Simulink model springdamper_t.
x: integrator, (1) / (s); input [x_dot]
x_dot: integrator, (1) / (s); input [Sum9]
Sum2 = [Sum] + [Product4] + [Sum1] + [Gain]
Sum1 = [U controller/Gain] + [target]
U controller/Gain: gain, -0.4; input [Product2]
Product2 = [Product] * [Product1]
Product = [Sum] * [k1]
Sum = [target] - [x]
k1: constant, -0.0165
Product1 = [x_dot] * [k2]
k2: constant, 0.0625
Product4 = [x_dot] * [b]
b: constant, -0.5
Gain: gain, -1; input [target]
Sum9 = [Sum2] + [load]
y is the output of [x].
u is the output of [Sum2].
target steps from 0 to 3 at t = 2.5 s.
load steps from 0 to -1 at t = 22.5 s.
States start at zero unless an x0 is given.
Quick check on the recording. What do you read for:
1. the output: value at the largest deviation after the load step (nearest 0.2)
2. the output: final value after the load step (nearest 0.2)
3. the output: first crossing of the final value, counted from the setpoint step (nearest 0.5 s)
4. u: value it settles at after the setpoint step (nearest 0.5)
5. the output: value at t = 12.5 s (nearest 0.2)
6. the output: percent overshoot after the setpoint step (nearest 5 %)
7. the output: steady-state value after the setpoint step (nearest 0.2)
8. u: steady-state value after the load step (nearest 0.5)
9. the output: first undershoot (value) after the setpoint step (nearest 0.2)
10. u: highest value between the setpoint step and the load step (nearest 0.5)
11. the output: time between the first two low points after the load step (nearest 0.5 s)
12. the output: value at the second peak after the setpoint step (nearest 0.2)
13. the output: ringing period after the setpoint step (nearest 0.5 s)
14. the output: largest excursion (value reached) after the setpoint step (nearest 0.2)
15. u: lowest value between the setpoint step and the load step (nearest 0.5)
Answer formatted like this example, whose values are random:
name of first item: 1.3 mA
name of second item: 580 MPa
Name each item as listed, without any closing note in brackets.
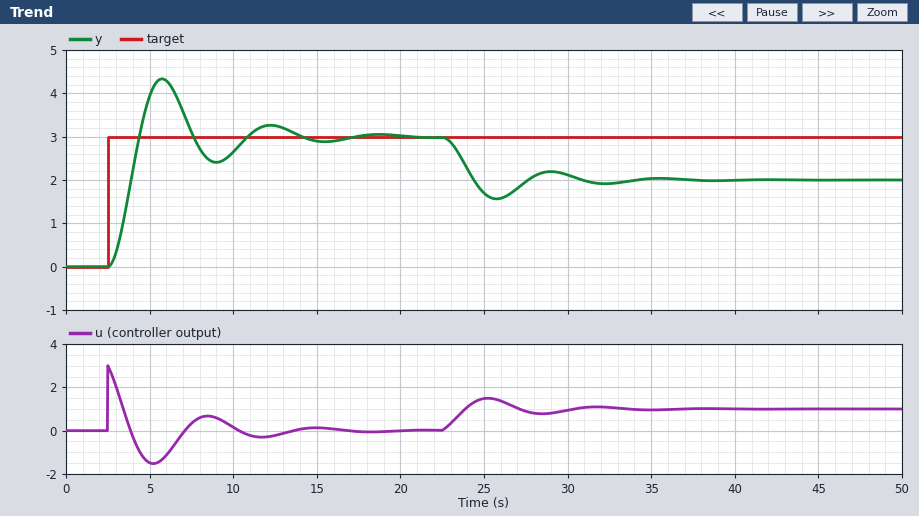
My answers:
the output: value at the largest deviation after the load step: 1.6
the output: final value after the load step: 2.0
the output: first crossing of the final value, counted from the setpoint step: 2.0 s
u: value it settles at after the setpoint step: 0.0
the output: value at t = 12.5 s: 3.2
the output: percent overshoot after the setpoint step: 45 %
the output: steady-state value after the setpoint step: 3.0
u: steady-state value after the load step: 1.0
the output: first undershoot (value) after the setpoint step: 2.4
u: highest value between the setpoint step and the load step: 3.0
the output: time between the first two low points after the load step: 6.5 s
the output: value at the second peak after the setpoint step: 3.2
the output: ringing period after the setpoint step: 6.5 s
the output: largest excursion (value reached) after the setpoint step: 4.4
u: lowest value between the setpoint step and the load step: -1.5
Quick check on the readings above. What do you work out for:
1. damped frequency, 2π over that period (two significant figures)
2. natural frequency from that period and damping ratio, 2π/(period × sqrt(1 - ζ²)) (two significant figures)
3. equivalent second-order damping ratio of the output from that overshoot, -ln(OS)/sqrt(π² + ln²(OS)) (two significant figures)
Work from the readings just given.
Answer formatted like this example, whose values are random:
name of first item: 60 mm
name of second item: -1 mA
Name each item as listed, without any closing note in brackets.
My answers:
damped frequency, 2π over that period: 0.97 rad/s
natural frequency from that period and damping ratio, 2π/(period × sqrt(1 - ζ²)): 1.00 rad/s
equivalent second-order damping ratio of the output from that overshoot, -ln(OS)/sqrt(π² + ln²(OS)): 0.25
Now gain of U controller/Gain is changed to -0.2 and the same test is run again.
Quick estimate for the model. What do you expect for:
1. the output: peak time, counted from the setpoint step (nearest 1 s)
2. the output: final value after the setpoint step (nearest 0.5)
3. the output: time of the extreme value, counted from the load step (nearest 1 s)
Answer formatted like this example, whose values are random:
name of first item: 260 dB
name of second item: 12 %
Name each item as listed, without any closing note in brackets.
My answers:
the output: peak time, counted from the setpoint step: 3 s
the output: final value after the setpoint step: 3.0
the output: time of the extreme value, counted from the load step: 3 s
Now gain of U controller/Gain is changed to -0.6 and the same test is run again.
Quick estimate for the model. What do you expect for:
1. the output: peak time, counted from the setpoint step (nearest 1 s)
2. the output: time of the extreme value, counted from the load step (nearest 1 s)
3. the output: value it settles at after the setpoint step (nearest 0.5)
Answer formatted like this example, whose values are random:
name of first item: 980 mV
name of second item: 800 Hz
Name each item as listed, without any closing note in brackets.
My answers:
the output: peak time, counted from the setpoint step: 3 s
the output: time of the extreme value, counted from the load step: 3 s
the output: value it settles at after the setpoint step: 3.0
